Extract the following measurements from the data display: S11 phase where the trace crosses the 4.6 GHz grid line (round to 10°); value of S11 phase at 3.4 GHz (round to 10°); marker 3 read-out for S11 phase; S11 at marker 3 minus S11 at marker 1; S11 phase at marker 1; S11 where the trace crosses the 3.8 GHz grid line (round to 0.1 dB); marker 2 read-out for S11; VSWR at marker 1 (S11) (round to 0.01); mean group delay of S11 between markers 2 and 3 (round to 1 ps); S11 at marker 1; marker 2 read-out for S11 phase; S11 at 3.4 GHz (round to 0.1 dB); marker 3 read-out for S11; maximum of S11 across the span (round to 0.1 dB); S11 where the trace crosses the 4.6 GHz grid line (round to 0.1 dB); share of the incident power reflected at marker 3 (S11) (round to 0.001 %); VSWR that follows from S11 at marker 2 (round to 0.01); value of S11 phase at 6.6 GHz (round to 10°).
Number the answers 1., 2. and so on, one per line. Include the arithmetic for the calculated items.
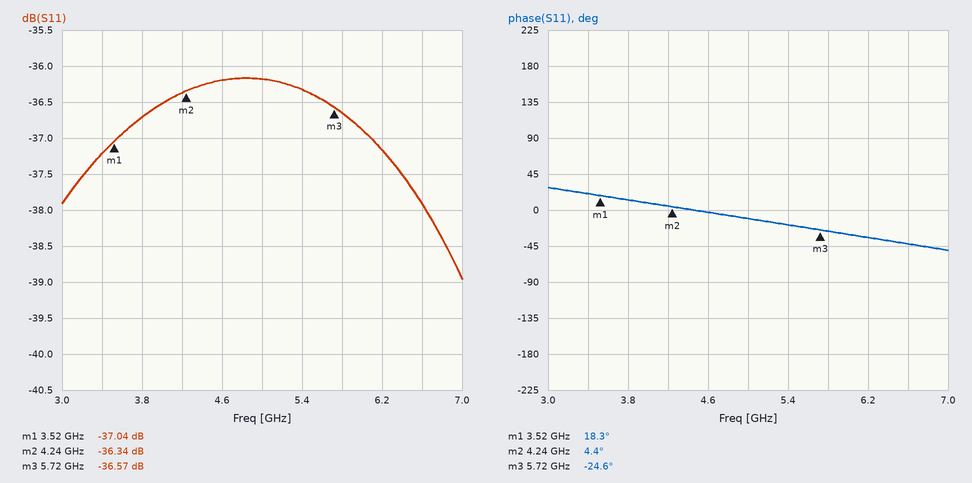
1. 0°
2. 20°
3. -24.6°
4. -36.57 − (-37.04) = 0.47 dB
5. 18.3°
6. -36.7 dB
7. -36.34 dB
8. (1 + 0.0141)/(1 − 0.0141) ≈ 1.03
9. −(-24.6° − (4.4°))/(360° × 1.48 GHz) ≈ 54 ps
10. -37.04 dB
11. 4.4°
12. -37.2 dB
13. -36.57 dB
14. -36.2 dB
15. -36.2 dB
16. 10^(-36.57/10) ≈ 0.022 %
17. (1 + 0.0152)/(1 − 0.0152) ≈ 1.03
18. -40°
